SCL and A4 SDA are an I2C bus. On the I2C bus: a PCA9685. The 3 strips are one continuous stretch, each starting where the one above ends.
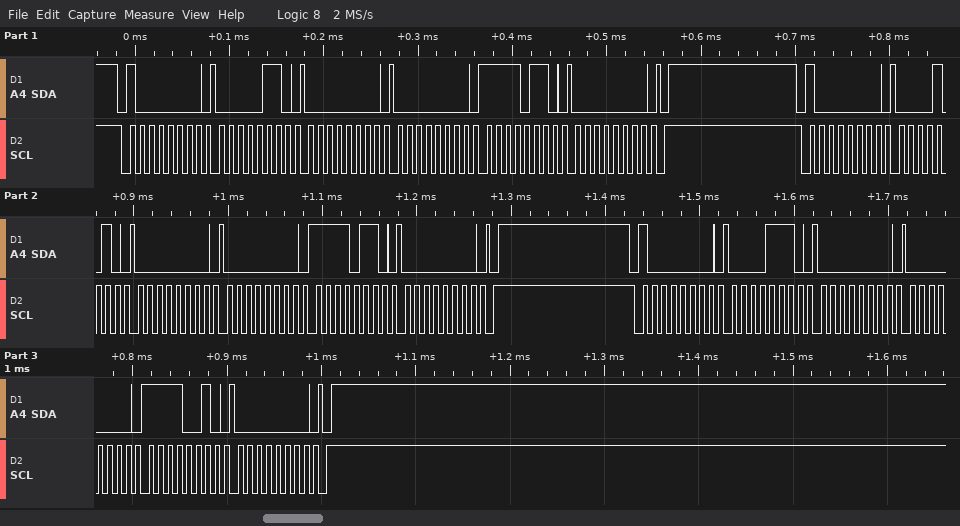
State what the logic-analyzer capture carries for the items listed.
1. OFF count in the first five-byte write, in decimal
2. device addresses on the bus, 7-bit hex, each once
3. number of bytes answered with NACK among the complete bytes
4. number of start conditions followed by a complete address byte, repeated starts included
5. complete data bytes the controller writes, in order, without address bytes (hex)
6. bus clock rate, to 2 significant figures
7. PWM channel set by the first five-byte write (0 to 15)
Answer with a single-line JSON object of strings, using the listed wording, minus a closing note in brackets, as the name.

{"OFF count in the first five-byte write, in decimal": "246", "device addresses on the bus, 7-bit hex, each once": "0x40", "number of bytes answered with NACK among the complete bytes": "0", "number of start conditions followed by a complete address byte, repeated starts included": "3", "complete data bytes the controller writes, in order, without address bytes": "06 00 00 F6 00 0A 00 00 F6 00 0E 00 00 F2 00", "bus clock rate, to 2 significant figures": "100 kHz", "PWM channel set by the first five-byte write": "0"}
